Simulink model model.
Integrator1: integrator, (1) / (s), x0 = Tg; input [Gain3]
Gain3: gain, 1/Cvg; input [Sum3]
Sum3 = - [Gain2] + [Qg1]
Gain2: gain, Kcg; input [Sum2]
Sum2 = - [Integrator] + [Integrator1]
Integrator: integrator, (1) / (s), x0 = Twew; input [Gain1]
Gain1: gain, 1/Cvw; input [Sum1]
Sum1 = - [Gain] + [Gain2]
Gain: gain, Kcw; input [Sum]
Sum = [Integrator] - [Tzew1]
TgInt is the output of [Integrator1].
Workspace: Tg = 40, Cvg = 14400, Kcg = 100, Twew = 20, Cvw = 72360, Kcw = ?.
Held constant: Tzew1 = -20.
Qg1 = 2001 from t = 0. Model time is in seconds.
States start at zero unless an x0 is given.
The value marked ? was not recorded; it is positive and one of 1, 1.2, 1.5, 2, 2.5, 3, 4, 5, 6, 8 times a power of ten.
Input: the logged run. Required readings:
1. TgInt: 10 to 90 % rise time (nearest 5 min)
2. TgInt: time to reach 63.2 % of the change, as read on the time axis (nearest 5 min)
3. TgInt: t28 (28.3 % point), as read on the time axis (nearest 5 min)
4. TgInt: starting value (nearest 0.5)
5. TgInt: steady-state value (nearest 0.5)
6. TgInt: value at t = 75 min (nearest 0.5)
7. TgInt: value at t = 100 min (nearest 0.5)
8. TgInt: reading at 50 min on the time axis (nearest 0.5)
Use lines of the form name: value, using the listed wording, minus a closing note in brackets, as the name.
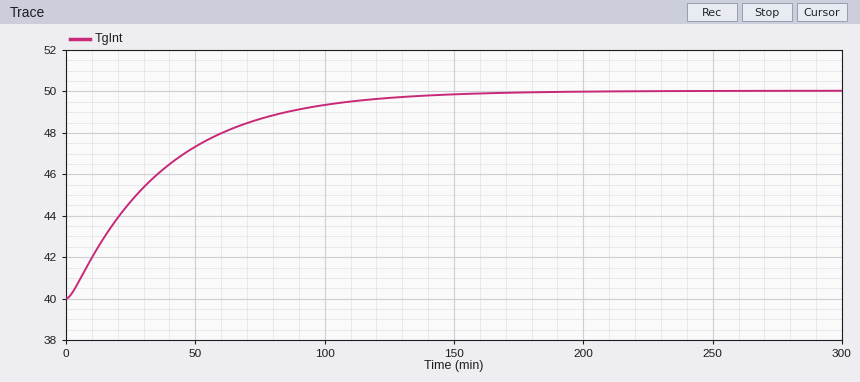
TgInt: 10 to 90 % rise time: 80 min
TgInt: time to reach 63.2 % of the change, as read on the time axis: 40 min
TgInt: t28 (28.3 % point), as read on the time axis: 15 min
TgInt: starting value: 40.0
TgInt: steady-state value: 50.0
TgInt: value at t = 75 min: 48.5
TgInt: value at t = 100 min: 49.5
TgInt: reading at 50 min on the time axis: 47.5
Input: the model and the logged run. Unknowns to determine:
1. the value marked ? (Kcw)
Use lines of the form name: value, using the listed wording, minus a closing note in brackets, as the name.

the value marked ?: 40
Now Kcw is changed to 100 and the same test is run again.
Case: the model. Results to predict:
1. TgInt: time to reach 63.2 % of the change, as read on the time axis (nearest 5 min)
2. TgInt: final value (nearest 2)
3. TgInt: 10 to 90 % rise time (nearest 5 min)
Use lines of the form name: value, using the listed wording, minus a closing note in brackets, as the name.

TgInt: time to reach 63.2 % of the change, as read on the time axis: 15 min
TgInt: final value: 20
TgInt: 10 to 90 % rise time: 35 min
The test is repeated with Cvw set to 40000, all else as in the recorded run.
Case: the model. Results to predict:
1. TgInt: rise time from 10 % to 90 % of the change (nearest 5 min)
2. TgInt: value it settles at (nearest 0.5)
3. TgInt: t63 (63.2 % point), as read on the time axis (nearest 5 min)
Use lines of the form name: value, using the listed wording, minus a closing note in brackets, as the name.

TgInt: rise time from 10 % to 90 % of the change: 50 min
TgInt: value it settles at: 50.0
TgInt: t63 (63.2 % point), as read on the time axis: 25 min
